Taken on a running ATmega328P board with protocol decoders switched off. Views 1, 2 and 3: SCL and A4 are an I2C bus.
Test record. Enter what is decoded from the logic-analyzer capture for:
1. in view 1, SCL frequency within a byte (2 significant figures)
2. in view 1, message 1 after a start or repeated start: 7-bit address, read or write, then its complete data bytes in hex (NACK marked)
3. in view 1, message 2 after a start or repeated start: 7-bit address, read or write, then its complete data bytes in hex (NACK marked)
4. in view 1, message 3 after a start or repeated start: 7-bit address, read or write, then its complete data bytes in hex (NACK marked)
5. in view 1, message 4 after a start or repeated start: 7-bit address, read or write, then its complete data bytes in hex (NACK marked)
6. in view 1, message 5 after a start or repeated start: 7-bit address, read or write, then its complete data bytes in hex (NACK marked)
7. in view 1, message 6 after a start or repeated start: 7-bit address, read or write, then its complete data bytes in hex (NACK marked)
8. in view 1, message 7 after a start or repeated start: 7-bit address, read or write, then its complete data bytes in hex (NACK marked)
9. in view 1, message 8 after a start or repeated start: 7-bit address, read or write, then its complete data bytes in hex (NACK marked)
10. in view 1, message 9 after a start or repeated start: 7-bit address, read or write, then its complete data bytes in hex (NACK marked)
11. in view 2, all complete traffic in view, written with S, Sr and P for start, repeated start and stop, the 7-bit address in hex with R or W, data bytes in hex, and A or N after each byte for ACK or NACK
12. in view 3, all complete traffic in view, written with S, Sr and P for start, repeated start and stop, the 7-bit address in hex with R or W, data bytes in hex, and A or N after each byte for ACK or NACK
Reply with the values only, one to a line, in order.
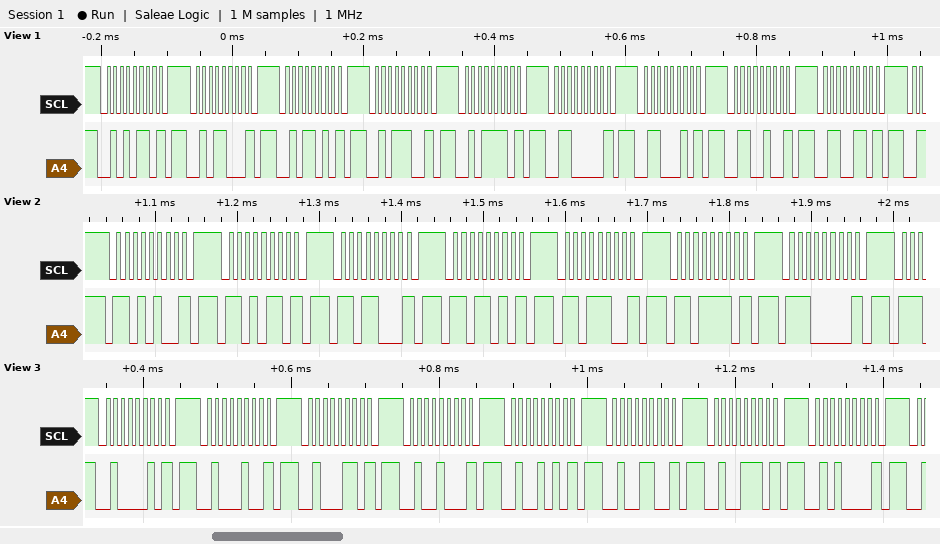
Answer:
100 kHz
0x2B write NACK
0x2C write NACK
0x2D write NACK
0x2E write NACK
0x2F write NACK
0x30 write NACK
0x31 write NACK
0x32 write NACK
0x33 write NACK
S 6AW N P S 6BW N P S 6CW N P S 6DW N P S 6EW N P S 6FW N P S 70W N P
S 21W N P S 22W N P S 23W N P S 24W N P S 25W N P S 26W N P S 27W N P S 28W N P
